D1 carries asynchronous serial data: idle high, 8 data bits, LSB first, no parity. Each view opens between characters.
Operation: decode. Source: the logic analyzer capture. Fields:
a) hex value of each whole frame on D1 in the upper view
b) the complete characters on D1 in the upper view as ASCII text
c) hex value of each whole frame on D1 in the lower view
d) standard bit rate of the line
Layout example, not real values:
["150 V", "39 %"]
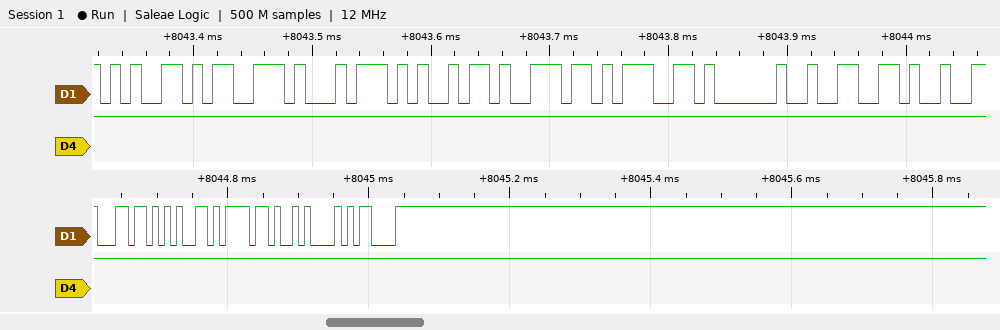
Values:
["65, 73, 74, 69, 6E, 67, 20, 66", "\"esting f\"", "6C, 65, 6F, 0A, 0D", "115200 baud"]
